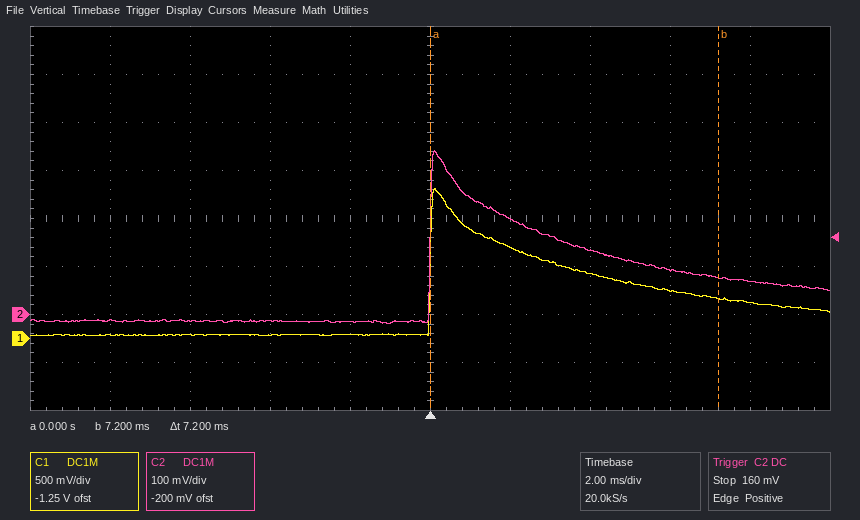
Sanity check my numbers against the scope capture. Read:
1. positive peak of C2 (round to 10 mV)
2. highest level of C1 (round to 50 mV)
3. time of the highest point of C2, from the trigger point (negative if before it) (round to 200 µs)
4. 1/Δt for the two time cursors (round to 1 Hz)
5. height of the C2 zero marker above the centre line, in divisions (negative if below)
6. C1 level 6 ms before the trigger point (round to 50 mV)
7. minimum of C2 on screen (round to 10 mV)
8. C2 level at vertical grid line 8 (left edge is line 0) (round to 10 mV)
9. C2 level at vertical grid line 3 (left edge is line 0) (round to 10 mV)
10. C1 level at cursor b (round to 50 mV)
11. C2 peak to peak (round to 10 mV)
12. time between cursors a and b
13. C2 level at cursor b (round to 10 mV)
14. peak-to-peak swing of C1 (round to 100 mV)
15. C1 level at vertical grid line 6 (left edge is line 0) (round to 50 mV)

340 mV
1.55 V
+200 µs
139 Hz
-2.0 div
50 mV
-20 mV
90 mV
-10 mV
400 mV
360 mV
7.2 ms
80 mV
1.50 V
950 mV
